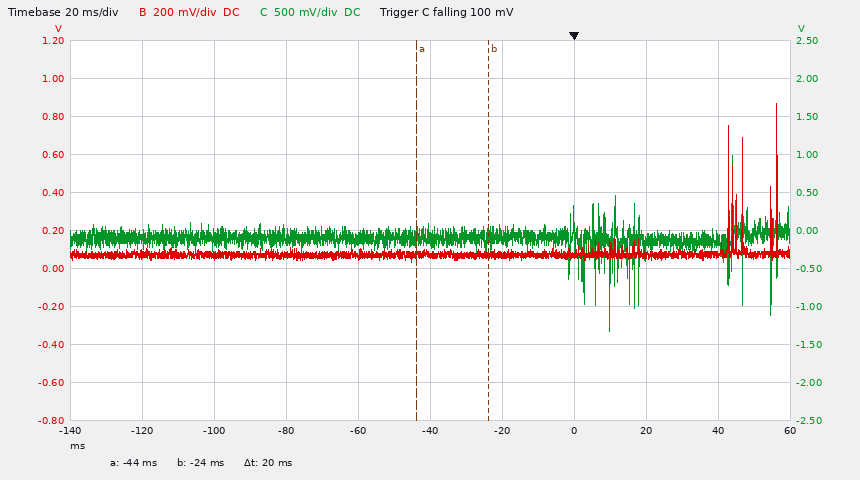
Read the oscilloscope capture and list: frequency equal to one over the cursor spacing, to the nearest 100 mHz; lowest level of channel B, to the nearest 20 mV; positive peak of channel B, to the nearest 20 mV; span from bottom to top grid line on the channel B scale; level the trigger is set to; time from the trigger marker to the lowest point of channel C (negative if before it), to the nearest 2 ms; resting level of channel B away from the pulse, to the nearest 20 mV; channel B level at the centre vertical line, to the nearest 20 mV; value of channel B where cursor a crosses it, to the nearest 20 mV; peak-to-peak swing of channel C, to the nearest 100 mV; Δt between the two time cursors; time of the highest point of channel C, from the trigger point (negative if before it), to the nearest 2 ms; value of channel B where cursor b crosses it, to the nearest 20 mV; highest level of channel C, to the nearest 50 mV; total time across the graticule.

50.0 Hz
40 mV
860 mV
2 V
100 mV
+10 ms
80 mV
80 mV
80 mV
2.30 V
20 ms
+44 ms
80 mV
1.00 V
200 ms
